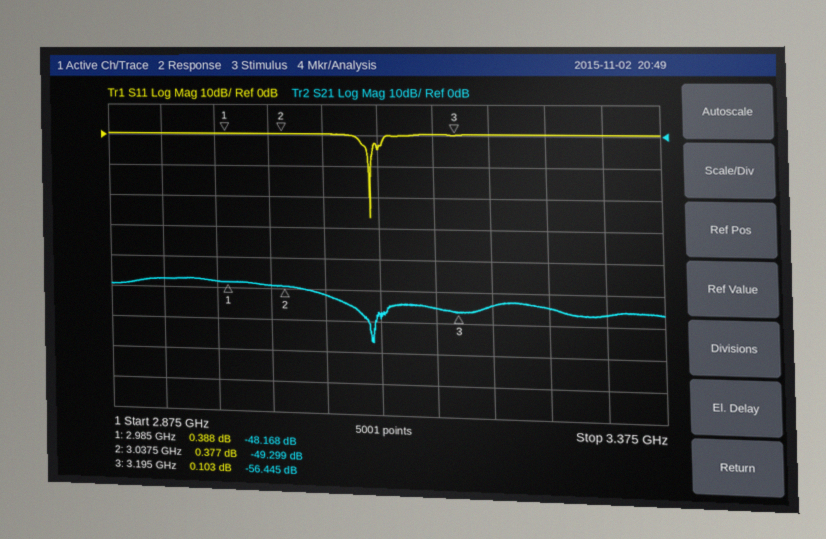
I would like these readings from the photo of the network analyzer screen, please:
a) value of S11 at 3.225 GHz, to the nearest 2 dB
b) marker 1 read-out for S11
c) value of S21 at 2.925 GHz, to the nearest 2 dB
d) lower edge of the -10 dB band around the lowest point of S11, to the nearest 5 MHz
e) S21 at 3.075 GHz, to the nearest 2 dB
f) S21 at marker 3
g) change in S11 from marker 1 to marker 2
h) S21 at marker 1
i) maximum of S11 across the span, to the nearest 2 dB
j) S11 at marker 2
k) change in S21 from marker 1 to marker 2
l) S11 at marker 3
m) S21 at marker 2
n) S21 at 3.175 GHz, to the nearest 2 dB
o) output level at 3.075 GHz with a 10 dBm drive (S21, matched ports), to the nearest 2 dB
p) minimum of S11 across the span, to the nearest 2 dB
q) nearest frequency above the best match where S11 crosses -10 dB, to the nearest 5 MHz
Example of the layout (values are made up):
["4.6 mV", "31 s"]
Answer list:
["0 dB", "0.388 dB", "-48 dB", "3.115 GHz", "-52 dB", "-56.445 dB", "-0.011 dB", "-48.168 dB", "0 dB", "0.377 dB", "-1.131 dB", "0.103 dB", "-49.299 dB", "-56 dB", "-42 dBm", "-26 dB", "3.120 GHz"]
